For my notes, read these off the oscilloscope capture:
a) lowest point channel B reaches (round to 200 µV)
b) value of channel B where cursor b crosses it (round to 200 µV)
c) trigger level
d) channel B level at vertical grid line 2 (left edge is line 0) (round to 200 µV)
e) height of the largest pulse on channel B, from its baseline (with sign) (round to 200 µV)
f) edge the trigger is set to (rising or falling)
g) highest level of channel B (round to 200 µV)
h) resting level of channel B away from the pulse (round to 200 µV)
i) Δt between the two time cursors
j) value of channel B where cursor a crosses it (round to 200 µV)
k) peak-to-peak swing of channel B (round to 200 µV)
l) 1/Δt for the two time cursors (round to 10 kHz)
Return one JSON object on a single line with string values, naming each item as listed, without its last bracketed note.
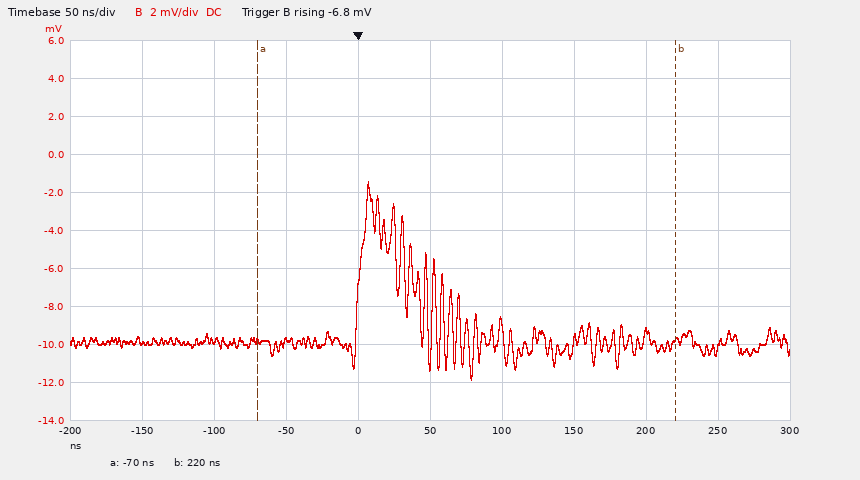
{"lowest point channel B reaches": "-11.8 mV", "value of channel B where cursor b crosses it": "-9.8 mV", "trigger level": "-6.8 mV", "channel B level at vertical grid line 2 (left edge is line 0)": "-9.8 mV", "height of the largest pulse on channel B, from its baseline (with sign)": "+8.4 mV", "edge the trigger is set to": "rising", "highest level of channel B": "-1.4 mV", "resting level of channel B away from the pulse": "-9.8 mV", "Δt between the two time cursors": "290 ns", "value of channel B where cursor a crosses it": "-9.8 mV", "peak-to-peak swing of channel B": "10.4 mV", "1/Δt for the two time cursors": "3.45 MHz"}
